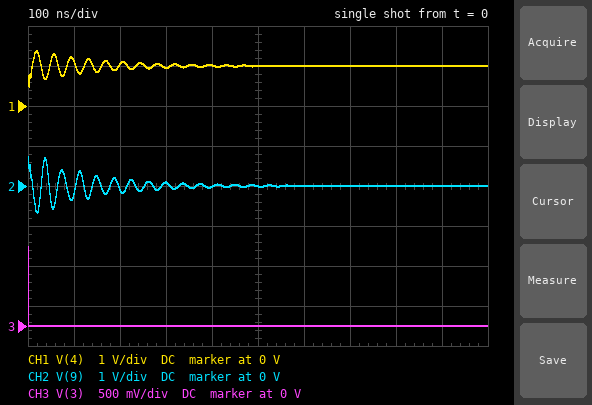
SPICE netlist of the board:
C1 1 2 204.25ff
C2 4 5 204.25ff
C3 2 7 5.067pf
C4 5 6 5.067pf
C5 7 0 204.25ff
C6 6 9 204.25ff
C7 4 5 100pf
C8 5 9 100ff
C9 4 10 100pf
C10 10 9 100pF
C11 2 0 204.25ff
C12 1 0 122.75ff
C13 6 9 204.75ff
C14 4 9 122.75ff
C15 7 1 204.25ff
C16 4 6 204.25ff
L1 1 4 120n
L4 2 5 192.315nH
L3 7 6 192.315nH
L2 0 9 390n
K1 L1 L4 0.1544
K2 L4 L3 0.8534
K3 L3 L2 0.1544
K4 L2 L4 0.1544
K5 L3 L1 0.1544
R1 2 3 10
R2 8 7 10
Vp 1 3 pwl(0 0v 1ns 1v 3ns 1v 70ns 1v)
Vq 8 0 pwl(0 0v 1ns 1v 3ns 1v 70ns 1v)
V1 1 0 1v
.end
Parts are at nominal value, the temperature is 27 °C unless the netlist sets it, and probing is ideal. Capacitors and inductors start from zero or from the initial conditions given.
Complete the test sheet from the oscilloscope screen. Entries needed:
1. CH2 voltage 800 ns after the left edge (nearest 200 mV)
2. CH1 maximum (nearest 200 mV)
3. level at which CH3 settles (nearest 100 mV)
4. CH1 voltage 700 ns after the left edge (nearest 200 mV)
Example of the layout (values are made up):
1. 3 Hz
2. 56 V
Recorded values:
1. 0 V
2. 1.4 V
3. 0 V
4. 1.0 V
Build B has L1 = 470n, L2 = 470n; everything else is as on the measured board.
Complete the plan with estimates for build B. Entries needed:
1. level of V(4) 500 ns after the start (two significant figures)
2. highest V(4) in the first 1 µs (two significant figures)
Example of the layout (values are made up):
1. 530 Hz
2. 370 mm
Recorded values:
1. 1.1 V
2. 1.7 V
